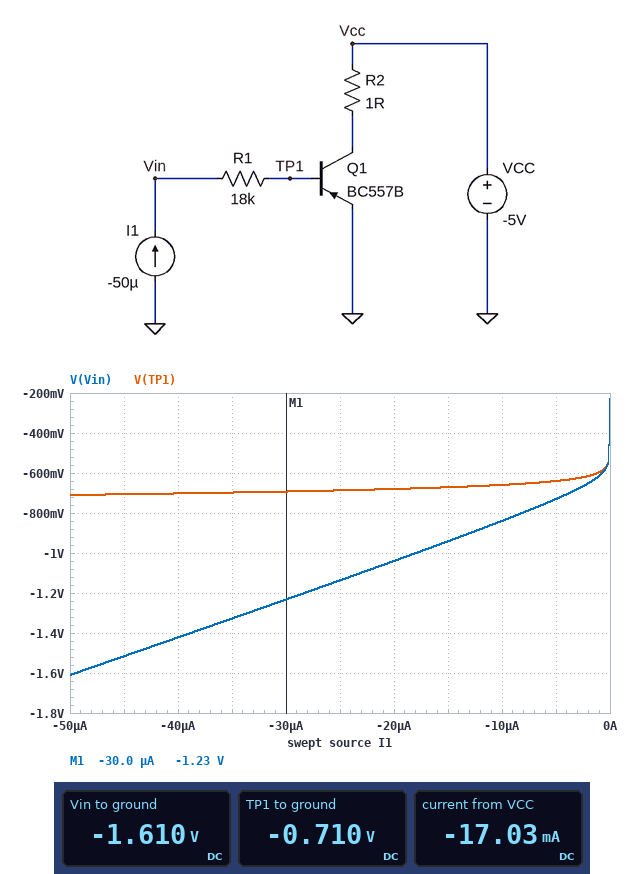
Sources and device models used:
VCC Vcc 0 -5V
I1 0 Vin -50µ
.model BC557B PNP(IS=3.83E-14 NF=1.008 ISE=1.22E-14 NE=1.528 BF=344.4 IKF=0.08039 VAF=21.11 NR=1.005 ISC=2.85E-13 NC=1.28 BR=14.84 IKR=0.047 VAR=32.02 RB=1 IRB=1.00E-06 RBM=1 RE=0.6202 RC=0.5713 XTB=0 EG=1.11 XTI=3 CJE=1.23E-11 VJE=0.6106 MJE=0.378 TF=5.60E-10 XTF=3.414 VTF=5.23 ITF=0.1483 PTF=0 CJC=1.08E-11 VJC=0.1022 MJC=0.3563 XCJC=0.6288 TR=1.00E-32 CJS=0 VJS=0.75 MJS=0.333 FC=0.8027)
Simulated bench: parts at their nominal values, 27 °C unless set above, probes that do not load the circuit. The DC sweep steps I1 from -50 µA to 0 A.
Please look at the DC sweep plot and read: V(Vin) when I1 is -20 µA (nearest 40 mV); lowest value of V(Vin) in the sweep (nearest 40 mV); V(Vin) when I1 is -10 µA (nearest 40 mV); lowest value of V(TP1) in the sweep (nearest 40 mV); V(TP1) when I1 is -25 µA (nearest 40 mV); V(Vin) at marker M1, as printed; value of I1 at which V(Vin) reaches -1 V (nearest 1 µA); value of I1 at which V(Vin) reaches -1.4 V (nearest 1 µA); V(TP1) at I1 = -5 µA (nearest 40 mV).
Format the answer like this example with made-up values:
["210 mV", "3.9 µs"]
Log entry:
["-1.04 V", "-1.60 V", "-840 mV", "-720 mV", "-680 mV", "-1.23 V", "-18 µA", "-39 µA", "-640 mV"]
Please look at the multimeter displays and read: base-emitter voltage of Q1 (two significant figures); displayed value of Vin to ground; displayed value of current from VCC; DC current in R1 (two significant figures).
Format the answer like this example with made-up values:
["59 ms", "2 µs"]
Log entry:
["-710 mV", "-1.610 V", "-17.03 mA", "50 µA"]
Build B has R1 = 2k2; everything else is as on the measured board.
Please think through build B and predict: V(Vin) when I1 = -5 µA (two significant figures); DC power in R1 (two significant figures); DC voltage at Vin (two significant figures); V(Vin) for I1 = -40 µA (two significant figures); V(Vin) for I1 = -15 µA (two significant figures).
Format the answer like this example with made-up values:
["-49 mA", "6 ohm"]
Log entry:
["-650 mV", "5.5 µW", "-820 mV", "-790 mV", "-700 mV"]
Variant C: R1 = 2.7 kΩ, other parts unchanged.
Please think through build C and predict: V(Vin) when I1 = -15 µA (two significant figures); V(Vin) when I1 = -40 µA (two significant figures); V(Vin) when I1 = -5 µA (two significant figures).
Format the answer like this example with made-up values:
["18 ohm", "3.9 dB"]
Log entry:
["-710 mV", "-810 mV", "-650 mV"]
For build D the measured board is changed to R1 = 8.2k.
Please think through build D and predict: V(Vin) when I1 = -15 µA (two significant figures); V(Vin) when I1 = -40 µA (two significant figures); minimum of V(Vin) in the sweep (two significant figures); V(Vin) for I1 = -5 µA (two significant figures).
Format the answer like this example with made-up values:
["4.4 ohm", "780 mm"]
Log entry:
["-790 mV", "-1.0 V", "-1.1 V", "-680 mV"]
